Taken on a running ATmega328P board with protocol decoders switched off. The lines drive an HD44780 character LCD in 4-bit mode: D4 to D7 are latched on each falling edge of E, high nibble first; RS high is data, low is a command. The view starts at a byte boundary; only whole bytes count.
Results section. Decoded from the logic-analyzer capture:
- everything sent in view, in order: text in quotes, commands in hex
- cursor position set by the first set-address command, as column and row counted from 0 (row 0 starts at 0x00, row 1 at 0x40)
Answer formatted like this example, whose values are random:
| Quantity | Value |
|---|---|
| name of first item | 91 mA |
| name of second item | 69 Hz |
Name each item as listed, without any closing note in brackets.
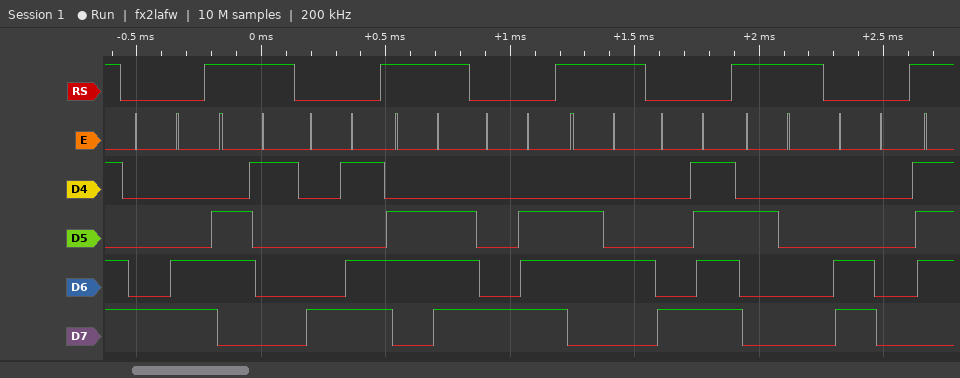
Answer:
| Quantity | Value |
|---|---|
| everything sent in view, in order: text in quotes, commands in hex | 0x8C "a" 0x8D "n" 0x8E "d" 0x8F " " 0xC0 |
| cursor position set by the first set-address command, as column and row counted from 0 | column 12, row 0 |
